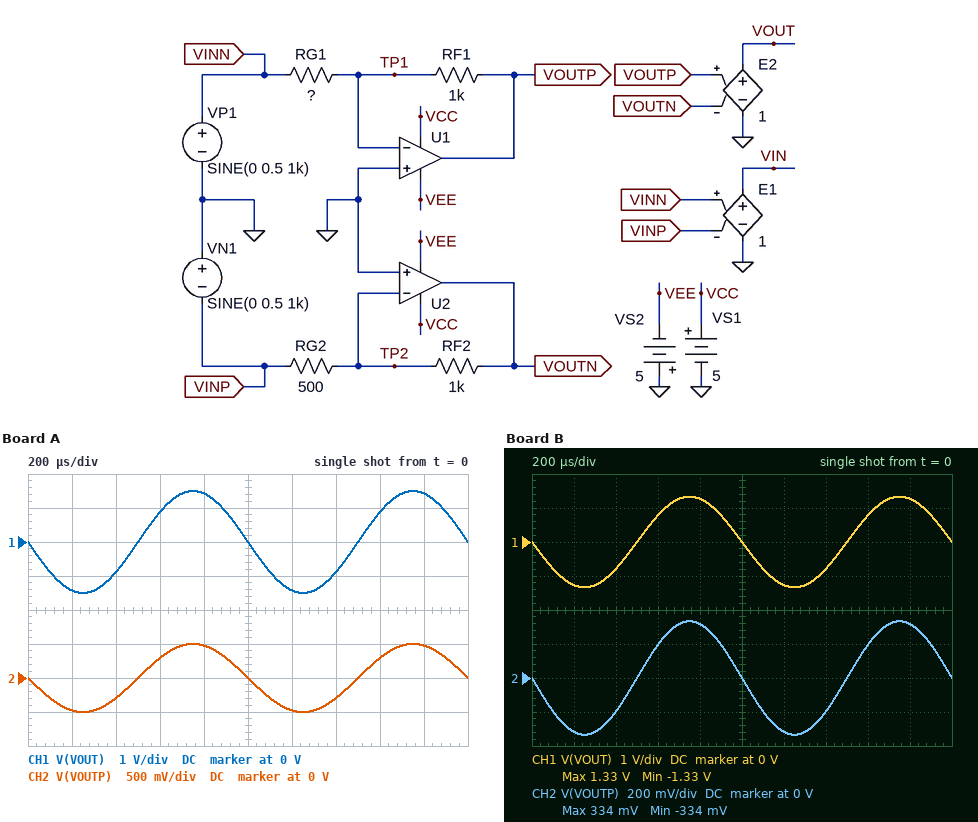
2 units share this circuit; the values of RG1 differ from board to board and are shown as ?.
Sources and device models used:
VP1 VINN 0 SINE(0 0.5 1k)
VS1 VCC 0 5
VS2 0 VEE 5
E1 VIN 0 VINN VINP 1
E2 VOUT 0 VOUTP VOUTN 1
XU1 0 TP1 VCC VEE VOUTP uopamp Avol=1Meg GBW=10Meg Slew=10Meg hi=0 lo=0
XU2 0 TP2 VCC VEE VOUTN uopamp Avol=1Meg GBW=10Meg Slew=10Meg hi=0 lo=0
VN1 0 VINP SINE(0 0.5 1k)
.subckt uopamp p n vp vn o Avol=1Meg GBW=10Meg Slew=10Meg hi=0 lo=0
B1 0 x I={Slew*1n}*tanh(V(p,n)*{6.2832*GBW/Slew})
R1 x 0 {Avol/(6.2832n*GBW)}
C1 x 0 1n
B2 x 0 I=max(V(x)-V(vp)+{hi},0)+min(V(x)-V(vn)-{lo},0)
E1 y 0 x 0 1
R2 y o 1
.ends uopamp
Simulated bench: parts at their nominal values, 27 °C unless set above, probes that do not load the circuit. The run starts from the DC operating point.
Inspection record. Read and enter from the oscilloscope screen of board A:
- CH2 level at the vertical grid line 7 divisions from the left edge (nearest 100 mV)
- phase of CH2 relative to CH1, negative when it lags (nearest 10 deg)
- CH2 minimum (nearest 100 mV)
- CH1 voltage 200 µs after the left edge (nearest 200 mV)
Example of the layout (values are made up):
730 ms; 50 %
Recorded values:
-300 mV; 0 deg; -500 mV; -1.4 V
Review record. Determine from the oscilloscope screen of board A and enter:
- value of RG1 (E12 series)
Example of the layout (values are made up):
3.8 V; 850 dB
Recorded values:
1 kΩ
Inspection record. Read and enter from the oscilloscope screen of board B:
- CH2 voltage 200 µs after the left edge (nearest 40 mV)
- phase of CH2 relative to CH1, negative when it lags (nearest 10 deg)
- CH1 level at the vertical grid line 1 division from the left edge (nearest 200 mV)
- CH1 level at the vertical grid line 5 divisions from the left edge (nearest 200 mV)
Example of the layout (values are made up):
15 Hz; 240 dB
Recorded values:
-320 mV; 0 deg; -1.2 V; 0 V
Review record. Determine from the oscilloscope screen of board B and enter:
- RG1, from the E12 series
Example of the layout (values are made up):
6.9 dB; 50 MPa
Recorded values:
1.5 kΩ
